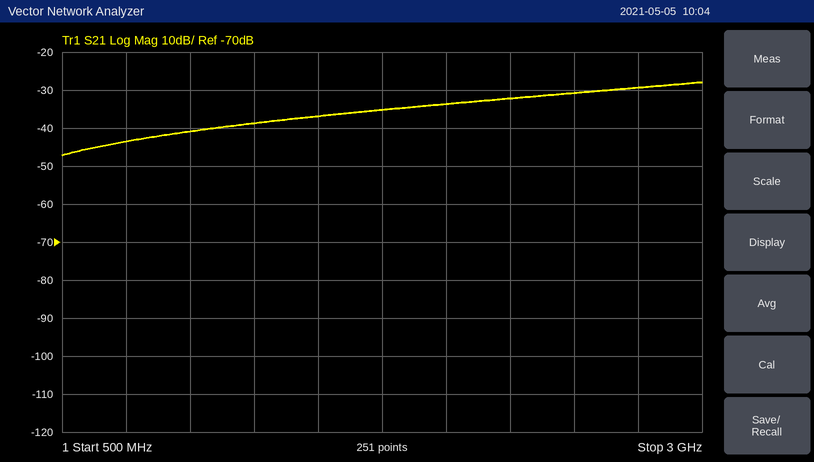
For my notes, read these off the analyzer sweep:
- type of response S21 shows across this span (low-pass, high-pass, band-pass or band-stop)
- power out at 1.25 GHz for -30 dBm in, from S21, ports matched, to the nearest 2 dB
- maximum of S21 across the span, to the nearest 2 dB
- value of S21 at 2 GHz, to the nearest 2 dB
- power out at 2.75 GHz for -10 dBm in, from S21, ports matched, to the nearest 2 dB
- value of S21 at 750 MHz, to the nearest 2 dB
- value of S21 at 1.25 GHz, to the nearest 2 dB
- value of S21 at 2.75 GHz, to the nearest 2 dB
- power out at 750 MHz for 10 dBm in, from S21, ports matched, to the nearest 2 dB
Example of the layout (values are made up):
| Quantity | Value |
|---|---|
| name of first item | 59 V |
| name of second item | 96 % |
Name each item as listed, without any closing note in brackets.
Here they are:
| Quantity | Value |
|---|---|
| type of response S21 shows across this span | high-pass |
| power out at 1.25 GHz for -30 dBm in, from S21, ports matched, to the nearest 2 dB | -68 dBm |
| maximum of S21 across the span, to the nearest 2 dB | -28 dB |
| value of S21 at 2 GHz, to the nearest 2 dB | -34 dB |
| power out at 2.75 GHz for -10 dBm in, from S21, ports matched, to the nearest 2 dB | -40 dBm |
| value of S21 at 750 MHz, to the nearest 2 dB | -44 dB |
| value of S21 at 1.25 GHz, to the nearest 2 dB | -38 dB |
| value of S21 at 2.75 GHz, to the nearest 2 dB | -30 dB |
| power out at 750 MHz for 10 dBm in, from S21, ports matched, to the nearest 2 dB | -34 dBm |
